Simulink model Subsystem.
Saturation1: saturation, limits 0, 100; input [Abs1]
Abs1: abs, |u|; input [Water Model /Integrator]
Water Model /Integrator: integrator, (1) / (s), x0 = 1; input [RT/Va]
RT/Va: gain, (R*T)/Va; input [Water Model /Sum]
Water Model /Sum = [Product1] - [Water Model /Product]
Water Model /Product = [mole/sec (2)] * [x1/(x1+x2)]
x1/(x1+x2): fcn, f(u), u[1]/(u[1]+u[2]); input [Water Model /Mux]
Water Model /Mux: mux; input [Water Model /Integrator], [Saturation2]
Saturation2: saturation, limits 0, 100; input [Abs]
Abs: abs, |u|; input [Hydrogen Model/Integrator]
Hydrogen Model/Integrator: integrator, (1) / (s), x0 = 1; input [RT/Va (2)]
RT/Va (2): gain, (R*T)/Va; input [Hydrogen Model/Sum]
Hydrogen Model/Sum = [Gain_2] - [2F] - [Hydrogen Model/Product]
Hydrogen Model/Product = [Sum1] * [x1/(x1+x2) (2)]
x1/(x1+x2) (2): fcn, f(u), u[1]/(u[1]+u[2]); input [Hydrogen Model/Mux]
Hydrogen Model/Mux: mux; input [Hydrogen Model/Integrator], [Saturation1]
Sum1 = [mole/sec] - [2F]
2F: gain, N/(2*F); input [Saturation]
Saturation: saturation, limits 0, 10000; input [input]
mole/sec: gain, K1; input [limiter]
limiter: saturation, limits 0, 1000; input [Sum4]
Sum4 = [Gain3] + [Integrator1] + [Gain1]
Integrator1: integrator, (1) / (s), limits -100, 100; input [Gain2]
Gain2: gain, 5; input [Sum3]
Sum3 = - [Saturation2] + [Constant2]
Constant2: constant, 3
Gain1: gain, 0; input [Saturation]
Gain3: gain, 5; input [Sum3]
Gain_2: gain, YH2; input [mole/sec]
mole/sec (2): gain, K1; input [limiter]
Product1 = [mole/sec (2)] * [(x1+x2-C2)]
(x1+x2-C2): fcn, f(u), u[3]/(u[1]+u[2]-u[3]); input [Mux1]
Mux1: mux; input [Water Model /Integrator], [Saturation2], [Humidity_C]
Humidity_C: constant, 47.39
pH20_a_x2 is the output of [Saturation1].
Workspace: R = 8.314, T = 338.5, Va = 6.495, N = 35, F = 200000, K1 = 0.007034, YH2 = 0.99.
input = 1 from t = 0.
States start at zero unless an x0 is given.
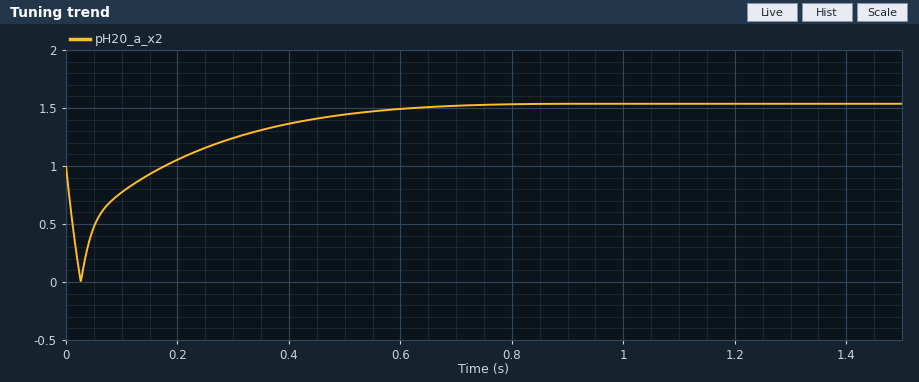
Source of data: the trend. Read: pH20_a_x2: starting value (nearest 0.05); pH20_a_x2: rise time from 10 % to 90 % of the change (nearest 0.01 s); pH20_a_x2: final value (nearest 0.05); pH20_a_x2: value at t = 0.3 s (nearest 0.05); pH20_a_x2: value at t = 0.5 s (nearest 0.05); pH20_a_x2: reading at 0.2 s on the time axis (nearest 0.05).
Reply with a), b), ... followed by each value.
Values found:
a) 1.00
b) 0.38 s
c) 1.55
d) 1.25
e) 1.45
f) 1.05
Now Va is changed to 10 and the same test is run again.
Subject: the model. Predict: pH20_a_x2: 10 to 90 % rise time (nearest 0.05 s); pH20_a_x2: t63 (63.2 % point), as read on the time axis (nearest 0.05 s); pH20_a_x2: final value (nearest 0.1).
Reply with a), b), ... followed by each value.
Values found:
a) 0.50 s
b) 0.55 s
c) 1.6
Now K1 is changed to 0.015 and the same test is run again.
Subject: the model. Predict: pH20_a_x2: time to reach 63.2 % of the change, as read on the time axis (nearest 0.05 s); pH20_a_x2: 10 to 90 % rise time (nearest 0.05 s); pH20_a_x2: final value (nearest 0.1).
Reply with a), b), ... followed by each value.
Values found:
a) 0.20 s
b) 0.20 s
c) 1.5
